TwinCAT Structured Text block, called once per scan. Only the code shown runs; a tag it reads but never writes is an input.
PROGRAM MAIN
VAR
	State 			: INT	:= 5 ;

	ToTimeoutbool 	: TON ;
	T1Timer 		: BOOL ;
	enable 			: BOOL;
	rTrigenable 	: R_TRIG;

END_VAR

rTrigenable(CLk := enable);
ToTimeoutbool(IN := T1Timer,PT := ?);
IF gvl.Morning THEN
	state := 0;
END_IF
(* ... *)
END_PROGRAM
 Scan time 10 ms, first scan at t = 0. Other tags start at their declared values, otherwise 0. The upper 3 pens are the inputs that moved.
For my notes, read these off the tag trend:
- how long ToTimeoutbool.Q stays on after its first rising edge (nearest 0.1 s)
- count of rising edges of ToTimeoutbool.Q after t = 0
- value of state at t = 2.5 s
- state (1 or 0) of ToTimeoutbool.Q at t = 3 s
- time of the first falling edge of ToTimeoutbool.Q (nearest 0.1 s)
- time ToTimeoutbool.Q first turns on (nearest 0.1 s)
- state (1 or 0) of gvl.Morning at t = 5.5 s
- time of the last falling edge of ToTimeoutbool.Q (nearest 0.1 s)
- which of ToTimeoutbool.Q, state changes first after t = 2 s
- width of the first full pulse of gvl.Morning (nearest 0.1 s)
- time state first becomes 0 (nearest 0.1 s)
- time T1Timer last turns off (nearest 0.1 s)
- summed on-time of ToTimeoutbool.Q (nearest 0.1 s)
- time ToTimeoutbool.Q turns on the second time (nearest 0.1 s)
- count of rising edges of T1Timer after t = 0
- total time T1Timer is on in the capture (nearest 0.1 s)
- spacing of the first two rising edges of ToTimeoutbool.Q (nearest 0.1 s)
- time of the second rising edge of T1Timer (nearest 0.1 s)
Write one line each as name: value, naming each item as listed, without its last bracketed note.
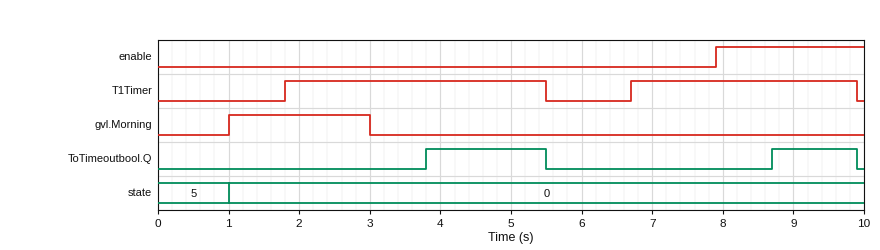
how long ToTimeoutbool.Q stays on after its first rising edge: 1.7 s
count of rising edges of ToTimeoutbool.Q after t = 0: 2
value of state at t = 2.5 s: 0
state (1 or 0) of ToTimeoutbool.Q at t = 3 s: 0
time of the first falling edge of ToTimeoutbool.Q: 5.5 s
time ToTimeoutbool.Q first turns on: 3.8 s
state (1 or 0) of gvl.Morning at t = 5.5 s: 0
time of the last falling edge of ToTimeoutbool.Q: 9.9 s
which of ToTimeoutbool.Q, state changes first after t = 2 s: ToTimeoutbool.Q
width of the first full pulse of gvl.Morning: 2.0 s
time state first becomes 0: 1.0 s
time T1Timer last turns off: 9.9 s
summed on-time of ToTimeoutbool.Q: 2.9 s
time ToTimeoutbool.Q turns on the second time: 8.7 s
count of rising edges of T1Timer after t = 0: 2
total time T1Timer is on in the capture: 6.9 s
spacing of the first two rising edges of ToTimeoutbool.Q: 4.9 s
time of the second rising edge of T1Timer: 6.7 s
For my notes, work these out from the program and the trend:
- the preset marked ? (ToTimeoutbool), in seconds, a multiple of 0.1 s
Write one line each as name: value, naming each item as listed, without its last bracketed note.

the preset marked ? (ToTimeoutbool), in seconds, a multiple of 0.1 s: 2.0 s
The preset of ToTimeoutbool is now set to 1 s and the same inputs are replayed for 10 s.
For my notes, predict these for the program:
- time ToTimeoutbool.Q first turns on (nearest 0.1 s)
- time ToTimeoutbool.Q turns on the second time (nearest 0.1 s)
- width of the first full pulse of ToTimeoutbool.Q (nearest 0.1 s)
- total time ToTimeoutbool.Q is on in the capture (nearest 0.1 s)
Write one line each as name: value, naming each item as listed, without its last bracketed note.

time ToTimeoutbool.Q first turns on: 2.8 s
time ToTimeoutbool.Q turns on the second time: 7.7 s
width of the first full pulse of ToTimeoutbool.Q: 2.7 s
total time ToTimeoutbool.Q is on in the capture: 4.9 s
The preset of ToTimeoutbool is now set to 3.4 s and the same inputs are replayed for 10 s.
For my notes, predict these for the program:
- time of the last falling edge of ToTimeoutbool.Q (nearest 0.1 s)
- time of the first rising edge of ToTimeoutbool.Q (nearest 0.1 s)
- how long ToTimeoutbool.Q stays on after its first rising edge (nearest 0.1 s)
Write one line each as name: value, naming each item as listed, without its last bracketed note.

time of the last falling edge of ToTimeoutbool.Q: 5.5 s
time of the first rising edge of ToTimeoutbool.Q: 5.2 s
how long ToTimeoutbool.Q stays on after its first rising edge: 0.3 s
